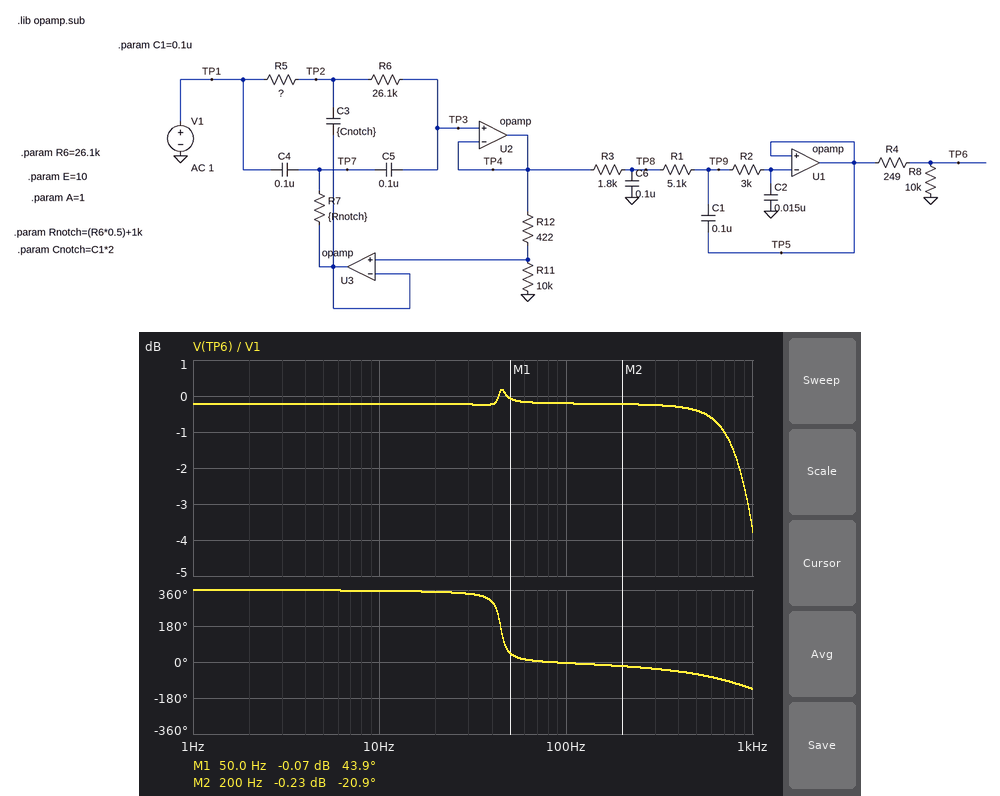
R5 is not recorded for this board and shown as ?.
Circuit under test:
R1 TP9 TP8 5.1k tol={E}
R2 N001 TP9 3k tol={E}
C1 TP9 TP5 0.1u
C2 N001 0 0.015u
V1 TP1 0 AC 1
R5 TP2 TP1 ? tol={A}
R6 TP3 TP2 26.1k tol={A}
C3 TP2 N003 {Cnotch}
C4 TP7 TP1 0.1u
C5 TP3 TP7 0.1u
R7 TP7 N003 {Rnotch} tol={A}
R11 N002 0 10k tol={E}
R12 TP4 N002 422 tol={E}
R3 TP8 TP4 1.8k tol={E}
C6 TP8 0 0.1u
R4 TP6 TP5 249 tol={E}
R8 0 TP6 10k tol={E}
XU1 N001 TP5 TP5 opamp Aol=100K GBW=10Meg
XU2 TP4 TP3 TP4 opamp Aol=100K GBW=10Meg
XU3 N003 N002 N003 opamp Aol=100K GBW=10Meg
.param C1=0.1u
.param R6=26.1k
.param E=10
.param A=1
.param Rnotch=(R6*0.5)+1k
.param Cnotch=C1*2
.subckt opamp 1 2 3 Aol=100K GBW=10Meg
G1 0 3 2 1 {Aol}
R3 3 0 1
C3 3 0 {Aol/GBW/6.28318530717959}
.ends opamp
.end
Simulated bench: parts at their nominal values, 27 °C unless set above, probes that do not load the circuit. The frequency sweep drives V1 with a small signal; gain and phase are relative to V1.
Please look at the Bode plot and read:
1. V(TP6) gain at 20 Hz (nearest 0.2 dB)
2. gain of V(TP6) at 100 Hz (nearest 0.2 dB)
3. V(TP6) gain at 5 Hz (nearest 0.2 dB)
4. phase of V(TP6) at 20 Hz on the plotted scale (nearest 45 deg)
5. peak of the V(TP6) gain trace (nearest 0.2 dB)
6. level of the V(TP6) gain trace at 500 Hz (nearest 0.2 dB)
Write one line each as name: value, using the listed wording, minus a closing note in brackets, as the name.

V(TP6) gain at 20 Hz: -0.2 dB
gain of V(TP6) at 100 Hz: -0.2 dB
V(TP6) gain at 5 Hz: -0.2 dB
phase of V(TP6) at 20 Hz on the plotted scale: 360 deg
peak of the V(TP6) gain trace: 0.2 dB
level of the V(TP6) gain trace at 500 Hz: -0.4 dB
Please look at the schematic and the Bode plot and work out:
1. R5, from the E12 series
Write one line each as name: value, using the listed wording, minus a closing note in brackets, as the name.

R5, from the E12 series: 56 kΩ
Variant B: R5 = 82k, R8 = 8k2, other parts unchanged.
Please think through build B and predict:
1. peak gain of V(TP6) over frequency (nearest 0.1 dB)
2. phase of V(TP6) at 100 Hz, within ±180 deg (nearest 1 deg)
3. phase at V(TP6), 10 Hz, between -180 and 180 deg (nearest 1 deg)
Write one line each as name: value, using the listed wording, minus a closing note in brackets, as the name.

peak gain of V(TP6) over frequency: 3.2 dB
phase of V(TP6) at 100 Hz, within ±180 deg: -5 deg
phase at V(TP6), 10 Hz, between -180 and 180 deg: -5 deg
